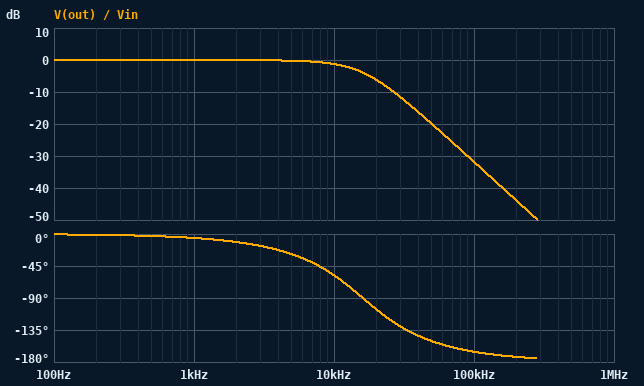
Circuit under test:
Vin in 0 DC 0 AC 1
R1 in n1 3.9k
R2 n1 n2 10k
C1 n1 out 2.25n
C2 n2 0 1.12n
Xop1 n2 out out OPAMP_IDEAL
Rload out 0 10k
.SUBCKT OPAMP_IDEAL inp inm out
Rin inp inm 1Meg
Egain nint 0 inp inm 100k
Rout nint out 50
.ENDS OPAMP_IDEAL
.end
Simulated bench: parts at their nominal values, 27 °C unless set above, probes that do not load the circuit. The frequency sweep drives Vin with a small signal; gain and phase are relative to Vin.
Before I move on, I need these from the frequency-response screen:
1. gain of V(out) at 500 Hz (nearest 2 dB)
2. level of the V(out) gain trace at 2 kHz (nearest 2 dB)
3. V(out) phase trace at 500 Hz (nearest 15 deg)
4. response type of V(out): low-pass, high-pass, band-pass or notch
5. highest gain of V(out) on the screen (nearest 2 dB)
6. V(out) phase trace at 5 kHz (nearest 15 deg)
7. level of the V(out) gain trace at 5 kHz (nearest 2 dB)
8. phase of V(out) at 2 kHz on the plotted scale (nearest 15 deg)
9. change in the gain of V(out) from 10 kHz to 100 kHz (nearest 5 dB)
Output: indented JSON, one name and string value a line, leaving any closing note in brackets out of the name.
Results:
{
  "gain of V(out) at 500 Hz": "0 dB",
  "level of the V(out) gain trace at 2 kHz": "0 dB",
  "V(out) phase trace at 500 Hz": "0 deg",
  "response type of V(out): low-pass, high-pass, band-pass or notch": "low-pass",
  "highest gain of V(out) on the screen": "0 dB",
  "V(out) phase trace at 5 kHz": "-30 deg",
  "level of the V(out) gain trace at 5 kHz": "0 dB",
  "phase of V(out) at 2 kHz on the plotted scale": "-15 deg",
  "change in the gain of V(out) from 10 kHz to 100 kHz": "-30 dB"
}
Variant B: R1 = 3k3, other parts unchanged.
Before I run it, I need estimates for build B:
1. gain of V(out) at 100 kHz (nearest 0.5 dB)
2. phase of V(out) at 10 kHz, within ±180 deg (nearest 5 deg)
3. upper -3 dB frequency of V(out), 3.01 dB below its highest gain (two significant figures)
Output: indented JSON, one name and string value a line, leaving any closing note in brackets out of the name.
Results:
{
  "gain of V(out) at 100 kHz": "-30.5 dB",
  "phase of V(out) at 10 kHz, within ±180 deg": "-55 deg",
  "upper -3 dB frequency of V(out), 3.01 dB below its highest gain": "15 kHz"
}
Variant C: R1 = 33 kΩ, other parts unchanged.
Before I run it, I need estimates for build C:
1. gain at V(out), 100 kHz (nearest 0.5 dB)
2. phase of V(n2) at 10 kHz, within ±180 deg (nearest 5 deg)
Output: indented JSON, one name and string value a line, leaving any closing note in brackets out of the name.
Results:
{
  "gain at V(out), 100 kHz": "-50.5 dB",
  "phase of V(n2) at 10 kHz, within ±180 deg": "-125 deg"
}
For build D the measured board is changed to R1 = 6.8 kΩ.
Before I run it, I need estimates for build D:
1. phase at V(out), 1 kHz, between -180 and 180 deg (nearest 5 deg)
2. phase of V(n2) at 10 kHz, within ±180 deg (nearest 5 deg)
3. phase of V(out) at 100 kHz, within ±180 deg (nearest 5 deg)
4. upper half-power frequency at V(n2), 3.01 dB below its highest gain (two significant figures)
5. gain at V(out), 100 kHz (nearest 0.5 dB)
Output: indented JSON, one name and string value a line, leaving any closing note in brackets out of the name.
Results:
{
  "phase at V(out), 1 kHz, between -180 and 180 deg": "-5 deg",
  "phase of V(n2) at 10 kHz, within ±180 deg": "-75 deg",
  "phase of V(out) at 100 kHz, within ±180 deg": "-170 deg",
  "upper half-power frequency at V(n2), 3.01 dB below its highest gain": "12 kHz",
  "gain at V(out), 100 kHz": "-36.5 dB"
}
